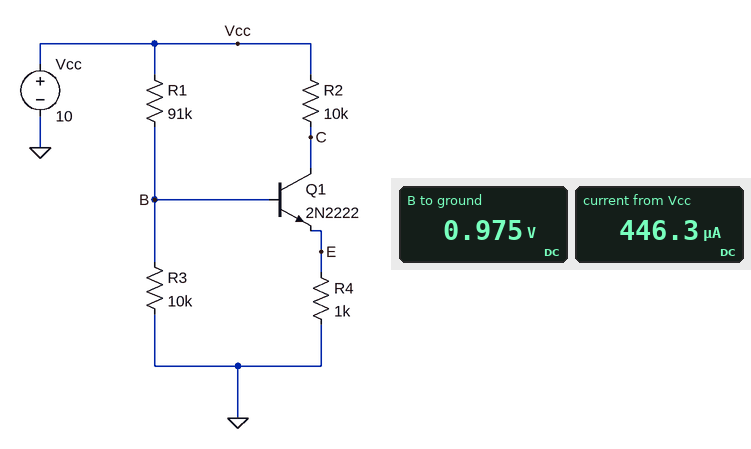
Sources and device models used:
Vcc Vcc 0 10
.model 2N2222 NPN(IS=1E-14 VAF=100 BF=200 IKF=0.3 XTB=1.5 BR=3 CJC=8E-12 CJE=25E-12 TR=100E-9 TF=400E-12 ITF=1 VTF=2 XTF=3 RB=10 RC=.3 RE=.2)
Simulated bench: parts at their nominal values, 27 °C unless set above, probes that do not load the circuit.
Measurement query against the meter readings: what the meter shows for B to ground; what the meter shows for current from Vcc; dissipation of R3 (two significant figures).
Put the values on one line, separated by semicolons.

0.975 V; 446.3 µA; 95 µW
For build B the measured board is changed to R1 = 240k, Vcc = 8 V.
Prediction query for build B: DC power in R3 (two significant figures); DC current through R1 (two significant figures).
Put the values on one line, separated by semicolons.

10 µW; 32 µA
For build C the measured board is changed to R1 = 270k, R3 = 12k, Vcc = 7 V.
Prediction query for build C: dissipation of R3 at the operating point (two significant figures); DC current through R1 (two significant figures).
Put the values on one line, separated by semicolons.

7.4 µW; 25 µA
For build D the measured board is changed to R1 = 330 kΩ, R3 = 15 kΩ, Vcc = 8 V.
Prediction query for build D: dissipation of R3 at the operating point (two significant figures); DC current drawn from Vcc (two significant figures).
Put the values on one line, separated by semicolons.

8.1 µW; 23 µA
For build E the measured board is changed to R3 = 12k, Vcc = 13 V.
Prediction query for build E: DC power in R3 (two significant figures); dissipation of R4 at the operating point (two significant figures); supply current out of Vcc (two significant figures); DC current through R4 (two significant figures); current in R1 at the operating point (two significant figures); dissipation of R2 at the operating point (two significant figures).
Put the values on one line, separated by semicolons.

180 µW; 680 µW; 950 µA; 820 µA; 130 µA; 6.7 mW
